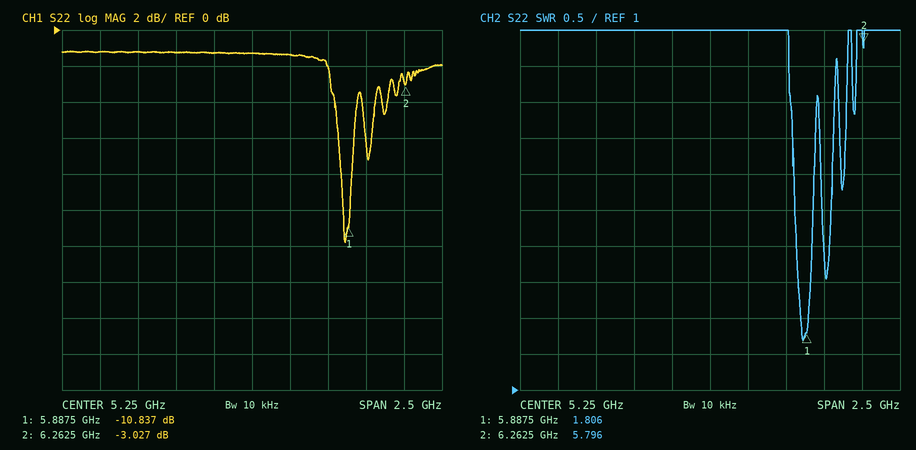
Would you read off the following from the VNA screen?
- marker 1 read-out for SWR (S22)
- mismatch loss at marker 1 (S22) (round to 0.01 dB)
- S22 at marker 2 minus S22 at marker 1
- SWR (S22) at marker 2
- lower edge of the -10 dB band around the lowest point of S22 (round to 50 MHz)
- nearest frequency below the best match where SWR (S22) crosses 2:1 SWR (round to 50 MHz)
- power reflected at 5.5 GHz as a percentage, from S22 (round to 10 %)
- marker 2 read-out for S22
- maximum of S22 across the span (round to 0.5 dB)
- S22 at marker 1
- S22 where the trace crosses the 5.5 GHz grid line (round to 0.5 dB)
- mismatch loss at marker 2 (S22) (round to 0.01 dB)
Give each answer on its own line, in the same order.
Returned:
1.806
0.37 dB
7.810 dB
5.796
5.85 GHz
5.85 GHz
70 %
-3.027 dB
-1.0 dB
-10.837 dB
-1.5 dB
2.99 dB
